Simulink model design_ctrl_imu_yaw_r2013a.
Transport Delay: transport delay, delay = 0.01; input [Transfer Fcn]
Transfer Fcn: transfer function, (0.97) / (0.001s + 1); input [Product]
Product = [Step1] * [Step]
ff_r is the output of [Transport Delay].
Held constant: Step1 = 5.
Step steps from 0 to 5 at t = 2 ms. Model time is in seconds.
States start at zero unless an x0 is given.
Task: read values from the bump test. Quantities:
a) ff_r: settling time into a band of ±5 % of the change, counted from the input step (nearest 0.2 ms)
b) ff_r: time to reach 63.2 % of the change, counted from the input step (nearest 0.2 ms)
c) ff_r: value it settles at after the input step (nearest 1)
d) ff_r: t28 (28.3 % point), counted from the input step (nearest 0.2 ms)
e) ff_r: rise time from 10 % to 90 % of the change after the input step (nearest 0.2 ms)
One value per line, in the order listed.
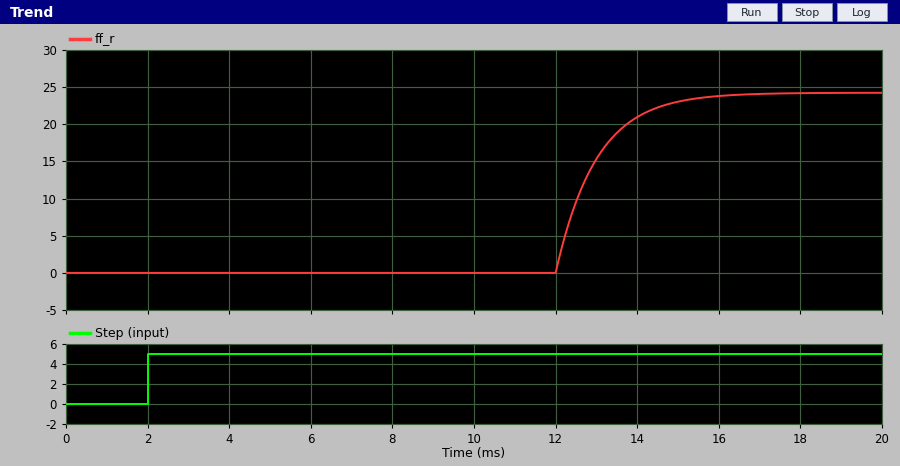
13.0 ms
11.0 ms
24
10.4 ms
2.2 ms
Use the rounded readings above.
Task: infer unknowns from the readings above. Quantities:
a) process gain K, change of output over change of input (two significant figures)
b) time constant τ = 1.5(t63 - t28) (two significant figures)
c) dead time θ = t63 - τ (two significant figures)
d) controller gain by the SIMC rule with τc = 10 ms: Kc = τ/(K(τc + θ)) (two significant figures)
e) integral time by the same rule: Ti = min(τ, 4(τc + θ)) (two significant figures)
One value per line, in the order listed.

4.8
0.90 ms
10 ms
0.0094
0.90 ms
